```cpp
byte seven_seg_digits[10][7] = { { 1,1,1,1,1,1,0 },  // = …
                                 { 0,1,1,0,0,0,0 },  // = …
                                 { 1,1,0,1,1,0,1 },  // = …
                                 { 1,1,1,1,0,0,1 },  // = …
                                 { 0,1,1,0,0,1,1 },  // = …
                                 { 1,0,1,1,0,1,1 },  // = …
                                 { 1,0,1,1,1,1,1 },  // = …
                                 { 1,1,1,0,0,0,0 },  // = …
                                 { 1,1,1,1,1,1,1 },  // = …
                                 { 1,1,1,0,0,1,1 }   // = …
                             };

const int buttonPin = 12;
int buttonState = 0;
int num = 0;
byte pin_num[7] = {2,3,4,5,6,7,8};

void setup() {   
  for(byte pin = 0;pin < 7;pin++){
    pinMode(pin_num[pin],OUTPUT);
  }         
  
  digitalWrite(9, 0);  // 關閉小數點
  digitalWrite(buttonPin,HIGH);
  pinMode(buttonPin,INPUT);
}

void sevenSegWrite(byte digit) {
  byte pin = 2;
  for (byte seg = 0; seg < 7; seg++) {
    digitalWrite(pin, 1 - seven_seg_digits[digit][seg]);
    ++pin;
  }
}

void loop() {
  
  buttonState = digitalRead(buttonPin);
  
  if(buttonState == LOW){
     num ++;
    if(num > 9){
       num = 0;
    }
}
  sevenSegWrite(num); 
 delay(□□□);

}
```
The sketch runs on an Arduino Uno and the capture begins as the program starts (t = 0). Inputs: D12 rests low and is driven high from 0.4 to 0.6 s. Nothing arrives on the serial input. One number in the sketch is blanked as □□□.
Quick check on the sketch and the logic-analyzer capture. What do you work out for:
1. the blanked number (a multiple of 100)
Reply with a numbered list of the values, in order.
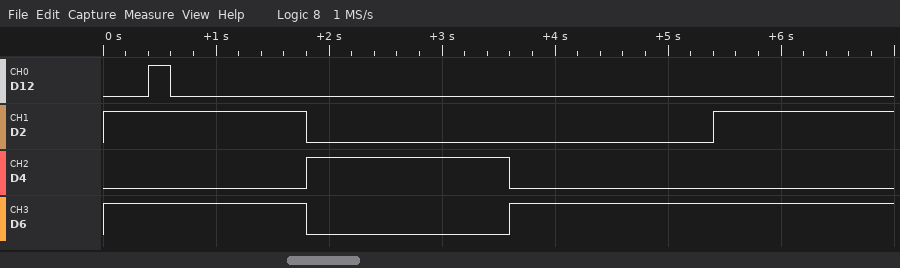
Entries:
1. 1800
